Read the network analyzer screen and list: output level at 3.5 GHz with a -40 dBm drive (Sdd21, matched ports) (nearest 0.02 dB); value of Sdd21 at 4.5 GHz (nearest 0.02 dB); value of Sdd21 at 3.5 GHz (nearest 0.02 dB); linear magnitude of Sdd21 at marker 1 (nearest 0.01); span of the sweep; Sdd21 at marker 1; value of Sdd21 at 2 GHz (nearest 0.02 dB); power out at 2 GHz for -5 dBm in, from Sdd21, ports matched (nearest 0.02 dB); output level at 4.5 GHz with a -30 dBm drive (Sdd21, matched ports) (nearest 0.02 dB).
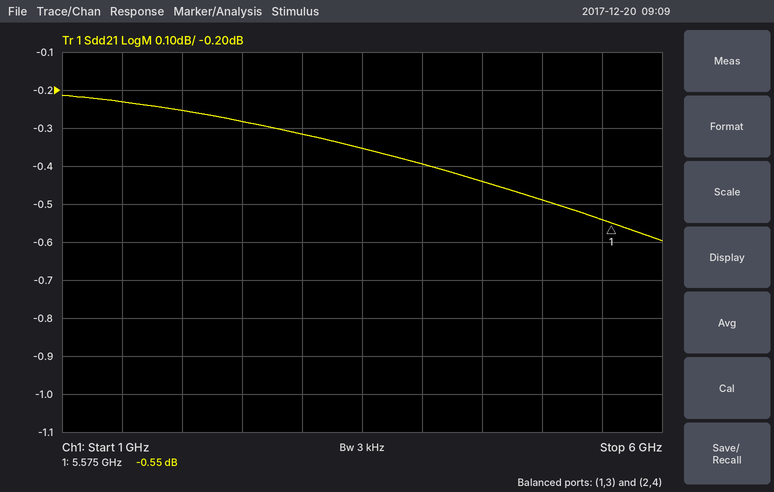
-40.36 dBm
-0.44 dB
-0.36 dB
0.94
5 GHz
-0.55 dB
-0.26 dB
-5.26 dBm
-30.44 dBm
